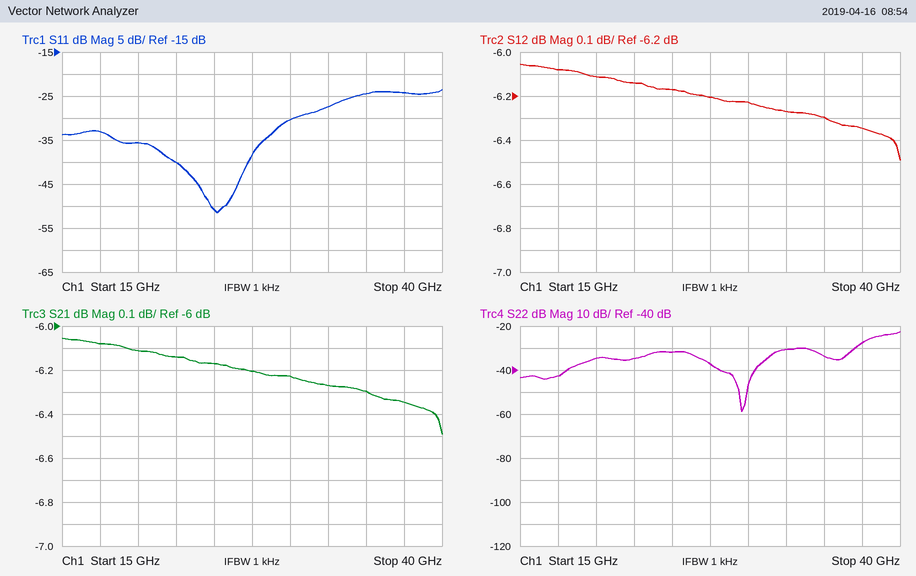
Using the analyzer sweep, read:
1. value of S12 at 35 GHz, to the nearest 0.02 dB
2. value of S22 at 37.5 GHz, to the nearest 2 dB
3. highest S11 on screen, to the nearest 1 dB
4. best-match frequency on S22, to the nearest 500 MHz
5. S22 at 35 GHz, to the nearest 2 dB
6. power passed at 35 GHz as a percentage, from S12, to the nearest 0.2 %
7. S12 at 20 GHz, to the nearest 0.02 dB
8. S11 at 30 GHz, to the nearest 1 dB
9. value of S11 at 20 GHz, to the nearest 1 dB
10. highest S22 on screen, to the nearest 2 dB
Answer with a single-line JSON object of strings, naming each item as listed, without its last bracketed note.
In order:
{"value of S12 at 35 GHz, to the nearest 0.02 dB": "-6.30 dB", "value of S22 at 37.5 GHz, to the nearest 2 dB": "-28 dB", "highest S11 on screen, to the nearest 1 dB": "-24 dB", "best-match frequency on S22, to the nearest 500 MHz": "29.5 GHz", "S22 at 35 GHz, to the nearest 2 dB": "-34 dB", "power passed at 35 GHz as a percentage, from S12, to the nearest 0.2 %": "23.4 %", "S12 at 20 GHz, to the nearest 0.02 dB": "-6.12 dB", "S11 at 30 GHz, to the nearest 1 dB": "-30 dB", "value of S11 at 20 GHz, to the nearest 1 dB": "-36 dB", "highest S22 on screen, to the nearest 2 dB": "-22 dB"}
